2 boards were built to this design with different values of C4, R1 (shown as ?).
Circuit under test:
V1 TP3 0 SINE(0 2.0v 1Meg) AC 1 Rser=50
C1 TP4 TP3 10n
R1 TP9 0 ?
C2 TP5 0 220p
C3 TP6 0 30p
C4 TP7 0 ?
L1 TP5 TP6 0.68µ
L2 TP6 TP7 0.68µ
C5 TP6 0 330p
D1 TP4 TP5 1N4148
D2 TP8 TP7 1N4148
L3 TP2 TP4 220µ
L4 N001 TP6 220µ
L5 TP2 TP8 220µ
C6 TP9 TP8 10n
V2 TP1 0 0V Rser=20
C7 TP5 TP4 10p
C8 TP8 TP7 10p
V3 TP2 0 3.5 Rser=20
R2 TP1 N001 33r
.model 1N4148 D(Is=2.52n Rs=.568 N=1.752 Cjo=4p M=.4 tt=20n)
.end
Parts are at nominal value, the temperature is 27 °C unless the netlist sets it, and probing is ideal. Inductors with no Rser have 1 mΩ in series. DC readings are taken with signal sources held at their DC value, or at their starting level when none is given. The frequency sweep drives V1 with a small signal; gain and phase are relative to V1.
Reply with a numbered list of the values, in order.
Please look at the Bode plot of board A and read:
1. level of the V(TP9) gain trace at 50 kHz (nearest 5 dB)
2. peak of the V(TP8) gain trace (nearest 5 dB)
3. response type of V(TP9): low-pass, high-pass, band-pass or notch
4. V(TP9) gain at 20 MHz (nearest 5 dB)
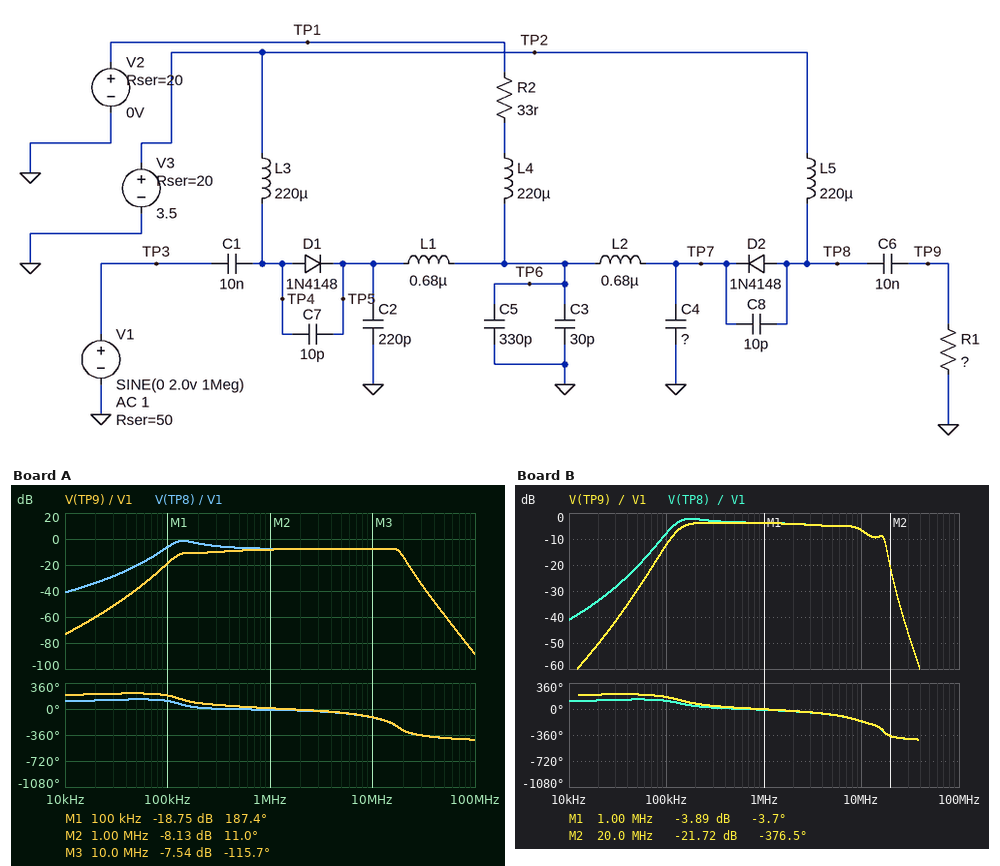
1. -40 dB
2. 0 dB
3. band-pass
4. -15 dB
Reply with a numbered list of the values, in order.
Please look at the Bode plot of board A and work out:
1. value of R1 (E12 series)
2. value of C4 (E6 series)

1. 39 Ω
2. 150 pF
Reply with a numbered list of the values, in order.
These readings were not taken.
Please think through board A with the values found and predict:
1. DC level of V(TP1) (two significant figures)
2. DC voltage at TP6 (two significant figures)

1. 760 mV
2. 2.0 V
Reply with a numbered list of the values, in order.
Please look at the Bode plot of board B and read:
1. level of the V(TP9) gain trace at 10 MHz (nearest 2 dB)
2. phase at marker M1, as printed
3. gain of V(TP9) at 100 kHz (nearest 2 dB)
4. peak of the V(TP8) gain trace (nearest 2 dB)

1. -6 dB
2. -3.7 deg
3. -12 dB
4. -2 dB
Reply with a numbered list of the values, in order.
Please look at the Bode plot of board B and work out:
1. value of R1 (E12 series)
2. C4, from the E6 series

1. 120 Ω
2. 680 pF
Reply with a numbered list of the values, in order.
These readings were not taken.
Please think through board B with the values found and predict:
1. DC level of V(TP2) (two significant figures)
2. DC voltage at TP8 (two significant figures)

1. 2.7 V
2. 2.7 V
